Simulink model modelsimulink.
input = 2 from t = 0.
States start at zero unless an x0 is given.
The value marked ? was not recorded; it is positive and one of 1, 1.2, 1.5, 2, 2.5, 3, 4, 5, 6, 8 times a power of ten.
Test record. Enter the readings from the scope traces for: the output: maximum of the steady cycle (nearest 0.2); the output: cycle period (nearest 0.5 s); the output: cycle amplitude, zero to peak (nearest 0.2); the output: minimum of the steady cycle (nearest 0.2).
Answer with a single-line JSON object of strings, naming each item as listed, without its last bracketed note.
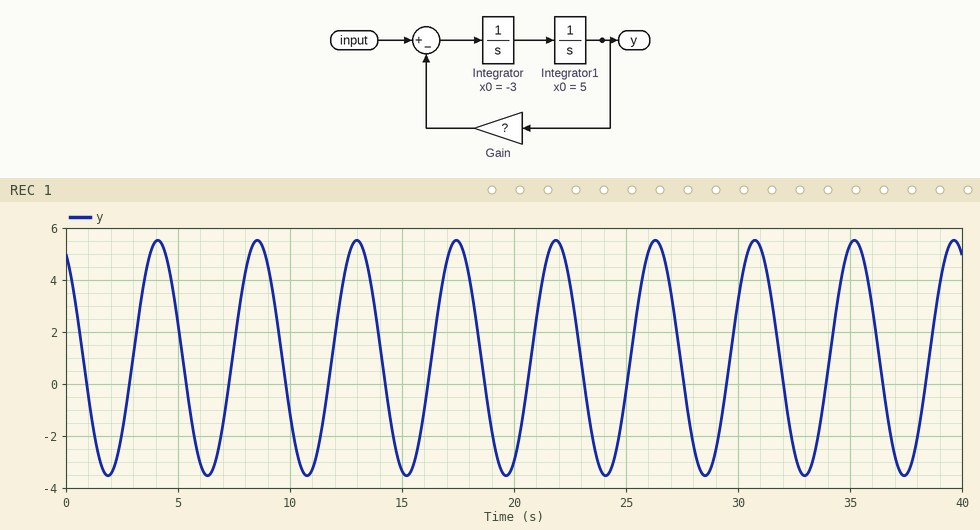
{"the output: maximum of the steady cycle": "5.6", "the output: cycle period": "4.5 s", "the output: cycle amplitude, zero to peak": "4.6", "the output: minimum of the steady cycle": "-3.6"}
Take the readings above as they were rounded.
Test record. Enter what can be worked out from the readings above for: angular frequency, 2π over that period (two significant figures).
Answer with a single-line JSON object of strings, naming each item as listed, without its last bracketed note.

{"angular frequency, 2π over that period": "1.4 rad/s"}
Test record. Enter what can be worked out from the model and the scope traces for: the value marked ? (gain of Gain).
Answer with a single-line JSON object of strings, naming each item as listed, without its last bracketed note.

{"the value marked ?": "2"}
